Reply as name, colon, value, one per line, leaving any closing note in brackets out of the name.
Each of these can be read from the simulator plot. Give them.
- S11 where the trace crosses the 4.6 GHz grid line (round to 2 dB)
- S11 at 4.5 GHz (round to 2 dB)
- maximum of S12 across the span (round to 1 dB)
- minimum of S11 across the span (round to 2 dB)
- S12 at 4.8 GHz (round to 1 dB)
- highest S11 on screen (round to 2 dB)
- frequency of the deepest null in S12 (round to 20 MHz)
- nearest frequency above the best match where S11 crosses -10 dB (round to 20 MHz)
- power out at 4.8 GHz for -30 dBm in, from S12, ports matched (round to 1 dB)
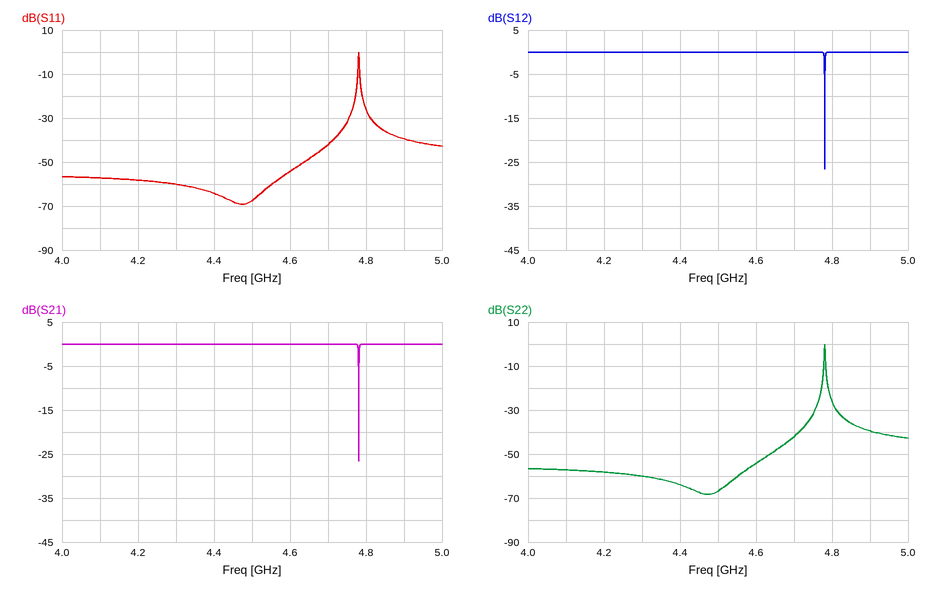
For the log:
S11 where the trace crosses the 4.6 GHz grid line: -54 dB
S11 at 4.5 GHz: -68 dB
maximum of S12 across the span: 0 dB
minimum of S11 across the span: -70 dB
S12 at 4.8 GHz: 0 dB
highest S11 on screen: 0 dB
frequency of the deepest null in S12: 4.78 GHz
nearest frequency above the best match where S11 crosses -10 dB: 4.78 GHz
power out at 4.8 GHz for -30 dBm in, from S12, ports matched: -30 dBm
